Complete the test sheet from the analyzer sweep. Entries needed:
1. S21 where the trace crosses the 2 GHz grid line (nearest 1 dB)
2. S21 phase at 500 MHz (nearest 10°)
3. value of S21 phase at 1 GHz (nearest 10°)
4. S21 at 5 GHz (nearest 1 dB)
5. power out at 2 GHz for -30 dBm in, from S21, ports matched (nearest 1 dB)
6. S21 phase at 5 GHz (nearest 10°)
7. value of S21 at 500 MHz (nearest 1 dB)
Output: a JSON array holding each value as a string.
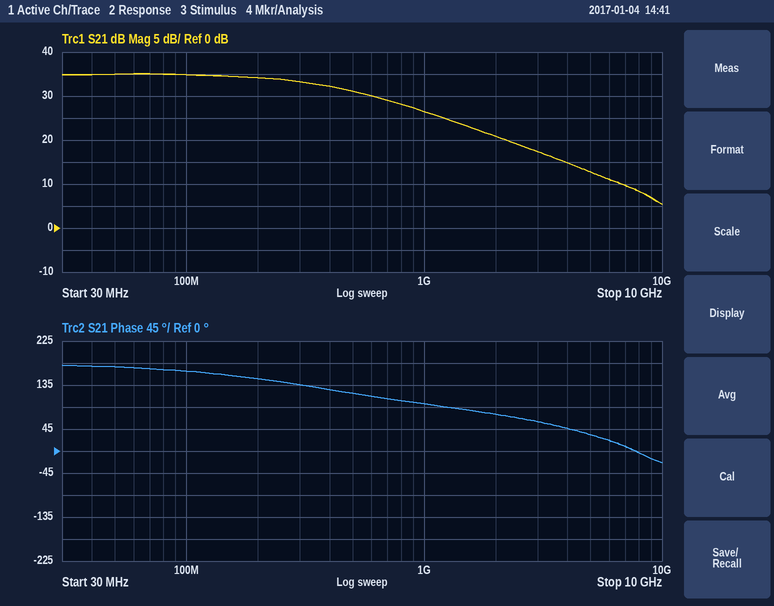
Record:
["21 dB", "120°", "100°", "13 dB", "-9 dBm", "30°", "31 dB"]
